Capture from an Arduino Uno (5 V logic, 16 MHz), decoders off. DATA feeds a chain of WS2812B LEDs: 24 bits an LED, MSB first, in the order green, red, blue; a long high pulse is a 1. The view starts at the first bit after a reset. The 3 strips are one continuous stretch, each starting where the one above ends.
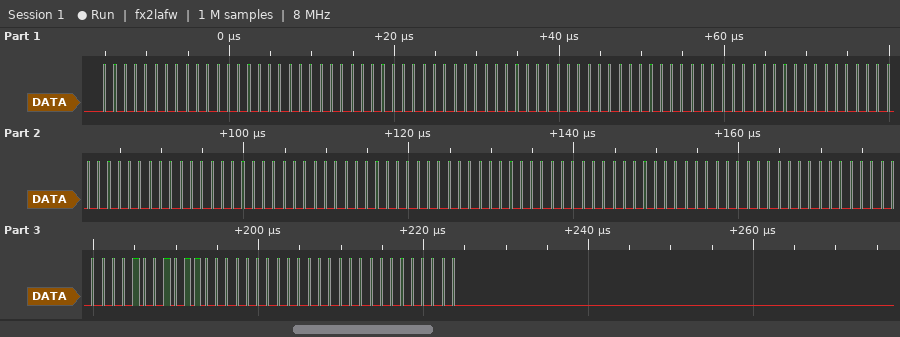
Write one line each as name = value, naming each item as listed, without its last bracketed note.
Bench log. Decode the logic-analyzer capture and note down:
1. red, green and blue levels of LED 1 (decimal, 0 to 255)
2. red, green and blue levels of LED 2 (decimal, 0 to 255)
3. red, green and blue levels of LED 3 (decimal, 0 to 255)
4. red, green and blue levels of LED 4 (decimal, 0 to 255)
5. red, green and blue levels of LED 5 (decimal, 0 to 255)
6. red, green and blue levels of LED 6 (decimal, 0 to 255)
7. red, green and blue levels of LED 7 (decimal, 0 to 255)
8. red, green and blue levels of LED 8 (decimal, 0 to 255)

red, green and blue levels of LED 1 = 0, 0, 0
red, green and blue levels of LED 2 = 0, 0, 0
red, green and blue levels of LED 3 = 0, 0, 0
red, green and blue levels of LED 4 = 0, 0, 0
red, green and blue levels of LED 5 = 0, 0, 0
red, green and blue levels of LED 6 = 0, 0, 0
red, green and blue levels of LED 7 = 0, 0, 150
red, green and blue levels of LED 8 = 0, 0, 0
